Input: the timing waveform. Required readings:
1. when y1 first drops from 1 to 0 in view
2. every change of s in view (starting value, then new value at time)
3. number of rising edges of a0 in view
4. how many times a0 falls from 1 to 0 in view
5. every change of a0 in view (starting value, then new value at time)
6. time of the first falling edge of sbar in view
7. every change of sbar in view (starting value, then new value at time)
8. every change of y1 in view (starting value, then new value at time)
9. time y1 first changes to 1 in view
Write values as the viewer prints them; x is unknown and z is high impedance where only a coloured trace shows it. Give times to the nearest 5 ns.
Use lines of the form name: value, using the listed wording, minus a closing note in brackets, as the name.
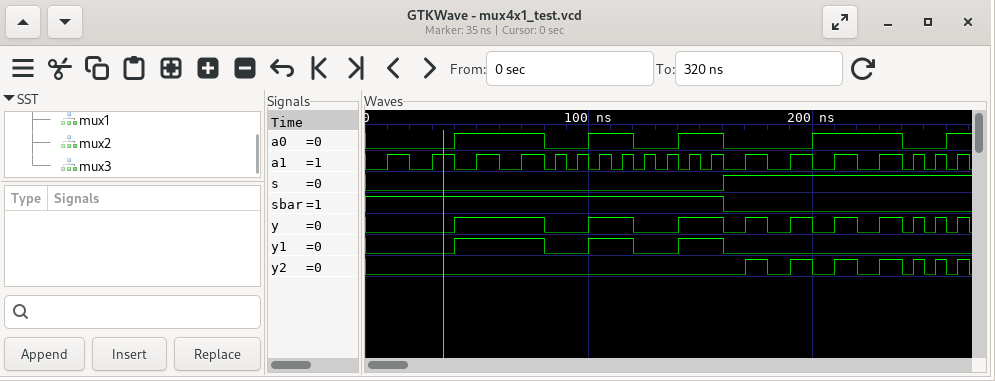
when y1 first drops from 1 to 0 in view: 80 ns
every change of s in view: 0, 1 at 160 ns
number of rising edges of a0 in view: 5
how many times a0 falls from 1 to 0 in view: 4
every change of a0 in view: 0, 1 at 40 ns, 0 at 80 ns, 1 at 100 ns, 0 at 120 ns, 1 at 140 ns, 0 at 160 ns, 1 at 200 ns, 0 at 240 ns, 1 at 260 ns
time of the first falling edge of sbar in view: 160 ns
every change of sbar in view: 1, 0 at 160 ns
every change of y1 in view: 0, 1 at 40 ns, 0 at 80 ns, 1 at 100 ns, 0 at 120 ns, 1 at 140 ns, 0 at 160 ns
time y1 first changes to 1 in view: 40 ns
